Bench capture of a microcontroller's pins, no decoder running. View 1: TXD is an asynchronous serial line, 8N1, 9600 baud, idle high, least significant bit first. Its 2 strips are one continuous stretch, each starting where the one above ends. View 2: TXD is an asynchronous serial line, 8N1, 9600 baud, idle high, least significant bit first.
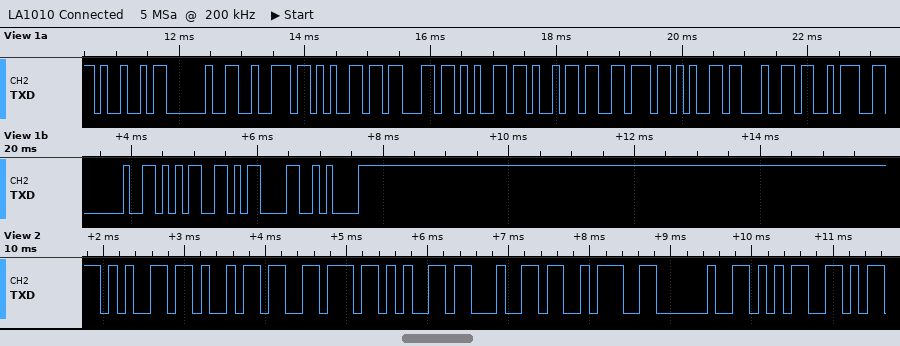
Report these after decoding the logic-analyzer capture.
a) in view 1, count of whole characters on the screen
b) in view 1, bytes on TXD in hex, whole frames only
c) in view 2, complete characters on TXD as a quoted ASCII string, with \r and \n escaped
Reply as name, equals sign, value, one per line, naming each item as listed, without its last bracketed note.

in view 1, count of whole characters on the screen = 15
in view 1, bytes on TXD in hex, whole frames only = 49 20 72 65 63 65 69 76 65 64 3A 20 35 0D 0A
in view 2, complete characters on TXD as a quoted ASCII string, with \r and \n escaped = "eived: 5"
